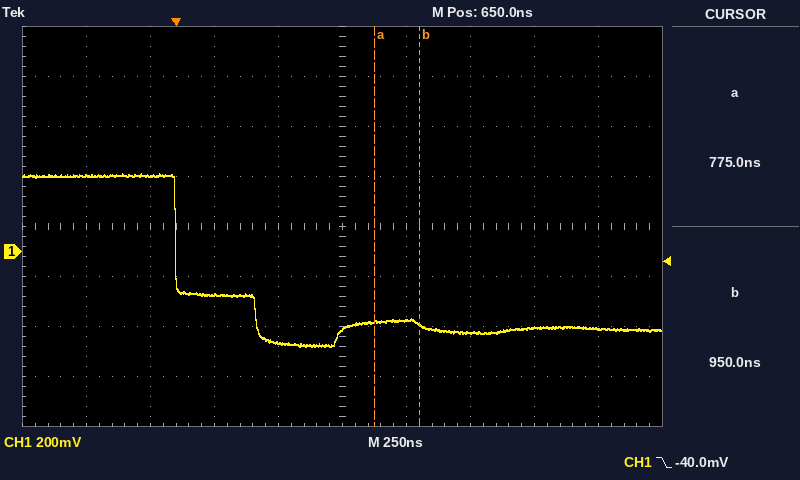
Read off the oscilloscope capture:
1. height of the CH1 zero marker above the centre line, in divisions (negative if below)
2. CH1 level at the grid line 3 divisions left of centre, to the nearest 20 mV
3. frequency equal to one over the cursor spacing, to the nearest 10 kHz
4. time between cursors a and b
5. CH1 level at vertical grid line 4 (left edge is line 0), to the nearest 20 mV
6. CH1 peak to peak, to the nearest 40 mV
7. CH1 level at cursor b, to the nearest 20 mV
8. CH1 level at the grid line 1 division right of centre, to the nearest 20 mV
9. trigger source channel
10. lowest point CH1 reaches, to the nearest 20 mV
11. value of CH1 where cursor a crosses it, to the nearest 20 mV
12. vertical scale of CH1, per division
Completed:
-0.5 div
300 mV
5.71 MHz
175 ns
-360 mV
680 mV
-300 mV
-280 mV
CH1
-380 mV
-280 mV
200 mV
